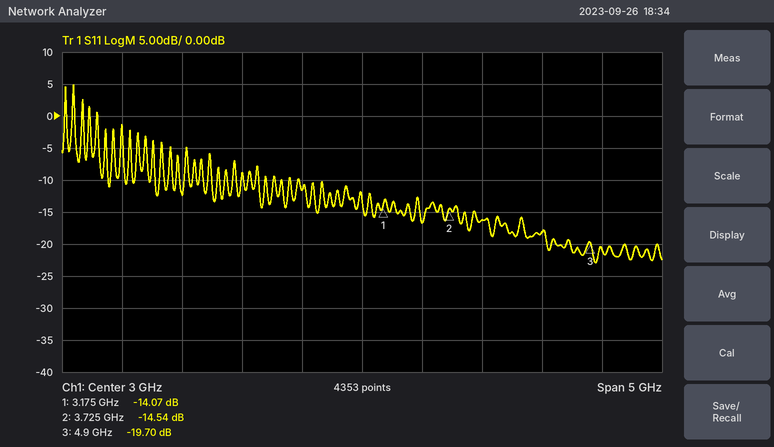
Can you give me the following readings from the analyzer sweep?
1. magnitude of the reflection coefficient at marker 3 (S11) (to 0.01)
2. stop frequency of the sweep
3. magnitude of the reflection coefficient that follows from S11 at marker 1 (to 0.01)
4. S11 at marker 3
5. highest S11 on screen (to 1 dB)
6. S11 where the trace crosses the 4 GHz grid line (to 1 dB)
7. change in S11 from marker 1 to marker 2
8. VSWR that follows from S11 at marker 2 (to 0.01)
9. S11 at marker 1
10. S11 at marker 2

0.10
5.5 GHz
0.20
-19.70 dB
5 dB
-16 dB
-0.47 dB
1.46
-14.07 dB
-14.54 dB
